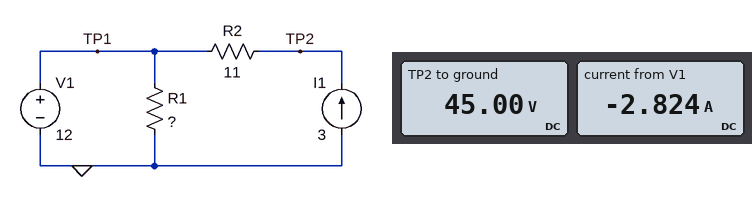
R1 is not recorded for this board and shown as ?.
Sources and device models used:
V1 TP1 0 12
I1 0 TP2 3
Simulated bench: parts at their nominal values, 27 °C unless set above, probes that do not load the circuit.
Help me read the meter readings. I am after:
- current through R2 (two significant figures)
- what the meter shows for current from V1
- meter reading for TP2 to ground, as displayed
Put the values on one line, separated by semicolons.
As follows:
3.0 A; -2.824 A; 45.00 V
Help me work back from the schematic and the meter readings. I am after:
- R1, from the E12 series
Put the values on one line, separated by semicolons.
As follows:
68 Ω
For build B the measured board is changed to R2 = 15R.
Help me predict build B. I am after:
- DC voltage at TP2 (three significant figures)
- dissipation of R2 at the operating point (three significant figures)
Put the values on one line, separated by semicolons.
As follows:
57.0 V; 135 W
